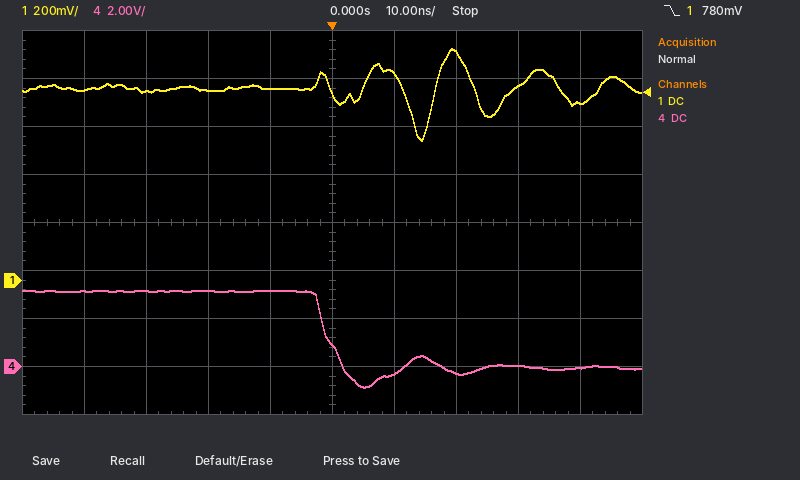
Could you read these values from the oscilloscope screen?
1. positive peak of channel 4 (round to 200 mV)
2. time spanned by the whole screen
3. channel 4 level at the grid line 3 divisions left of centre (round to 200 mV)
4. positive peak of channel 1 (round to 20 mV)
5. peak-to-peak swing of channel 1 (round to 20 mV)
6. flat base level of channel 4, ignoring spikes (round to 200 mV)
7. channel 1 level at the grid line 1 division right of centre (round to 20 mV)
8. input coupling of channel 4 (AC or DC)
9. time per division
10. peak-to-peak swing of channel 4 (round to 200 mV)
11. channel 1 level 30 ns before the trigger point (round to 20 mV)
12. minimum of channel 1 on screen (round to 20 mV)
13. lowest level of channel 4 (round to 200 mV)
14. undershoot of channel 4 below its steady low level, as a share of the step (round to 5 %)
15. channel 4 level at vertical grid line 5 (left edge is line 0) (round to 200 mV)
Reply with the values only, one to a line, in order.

3.2 V
100 ns
3.2 V
960 mV
380 mV
0.0 V
860 mV
DC
10 ns
4.0 V
780 mV
580 mV
-800 mV
25 %
1.0 V
